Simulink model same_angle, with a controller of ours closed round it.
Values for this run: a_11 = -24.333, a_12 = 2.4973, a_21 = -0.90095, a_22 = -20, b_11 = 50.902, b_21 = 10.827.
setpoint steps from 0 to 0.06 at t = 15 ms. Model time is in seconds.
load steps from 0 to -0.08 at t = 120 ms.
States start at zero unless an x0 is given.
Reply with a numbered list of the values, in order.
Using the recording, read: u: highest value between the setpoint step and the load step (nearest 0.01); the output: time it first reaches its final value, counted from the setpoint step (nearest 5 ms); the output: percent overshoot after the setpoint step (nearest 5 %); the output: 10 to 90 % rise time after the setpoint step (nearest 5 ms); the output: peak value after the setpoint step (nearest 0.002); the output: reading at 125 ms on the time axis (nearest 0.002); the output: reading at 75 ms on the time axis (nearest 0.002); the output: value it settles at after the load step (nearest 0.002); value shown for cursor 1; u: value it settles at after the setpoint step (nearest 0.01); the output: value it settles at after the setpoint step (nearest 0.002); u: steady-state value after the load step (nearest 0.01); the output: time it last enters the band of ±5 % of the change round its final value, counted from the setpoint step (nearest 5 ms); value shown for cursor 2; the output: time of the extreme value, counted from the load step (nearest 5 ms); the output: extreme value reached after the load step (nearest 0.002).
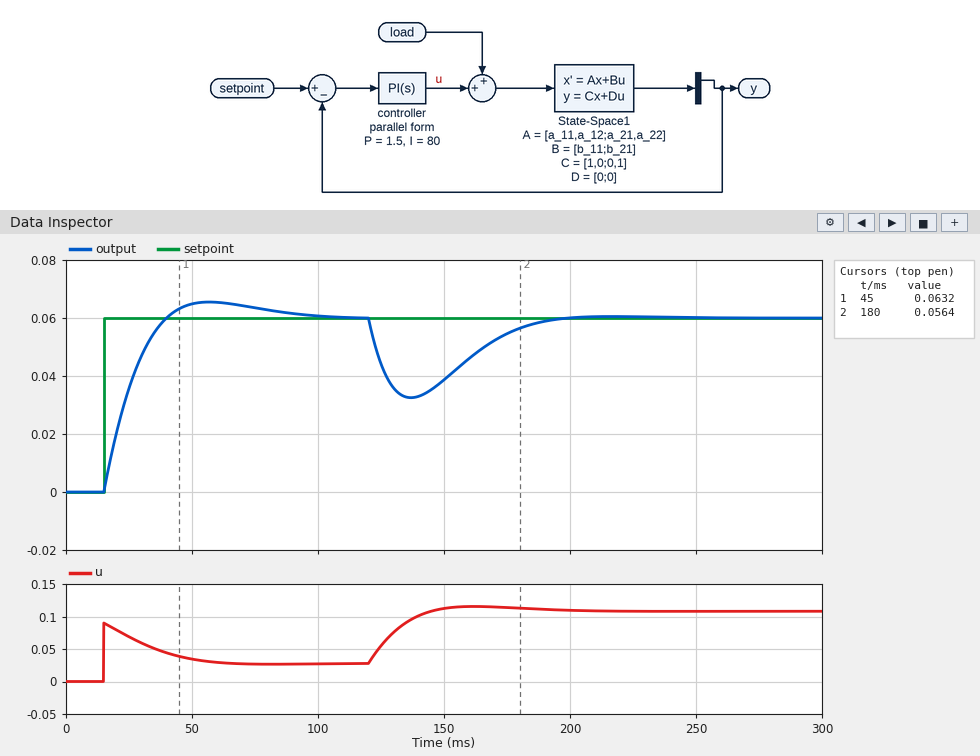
1. 0.09
2. 25 ms
3. 10 %
4. 20 ms
5. 0.066
6. 0.044
7. 0.064
8. 0.060
9. 0.0632
10. 0.03
11. 0.060
12. 0.11
13. 65 ms
14. 0.0564
15. 15 ms
16. 0.032
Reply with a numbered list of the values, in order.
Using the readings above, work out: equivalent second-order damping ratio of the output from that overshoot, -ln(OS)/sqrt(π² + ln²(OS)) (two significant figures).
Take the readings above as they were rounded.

1. 0.59
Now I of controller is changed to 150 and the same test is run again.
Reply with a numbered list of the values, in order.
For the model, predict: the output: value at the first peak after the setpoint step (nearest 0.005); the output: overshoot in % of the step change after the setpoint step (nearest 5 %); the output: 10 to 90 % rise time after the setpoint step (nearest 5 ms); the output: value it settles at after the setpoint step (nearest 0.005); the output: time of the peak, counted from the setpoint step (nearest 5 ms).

1. 0.070
2. 20 %
3. 15 ms
4. 0.060
5. 30 ms
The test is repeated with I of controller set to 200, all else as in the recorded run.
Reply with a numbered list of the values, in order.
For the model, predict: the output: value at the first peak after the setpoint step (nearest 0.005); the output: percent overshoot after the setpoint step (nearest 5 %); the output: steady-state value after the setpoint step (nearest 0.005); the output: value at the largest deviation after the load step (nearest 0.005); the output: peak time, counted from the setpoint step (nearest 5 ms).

1. 0.075
2. 25 %
3. 0.060
4. 0.040
5. 25 ms
